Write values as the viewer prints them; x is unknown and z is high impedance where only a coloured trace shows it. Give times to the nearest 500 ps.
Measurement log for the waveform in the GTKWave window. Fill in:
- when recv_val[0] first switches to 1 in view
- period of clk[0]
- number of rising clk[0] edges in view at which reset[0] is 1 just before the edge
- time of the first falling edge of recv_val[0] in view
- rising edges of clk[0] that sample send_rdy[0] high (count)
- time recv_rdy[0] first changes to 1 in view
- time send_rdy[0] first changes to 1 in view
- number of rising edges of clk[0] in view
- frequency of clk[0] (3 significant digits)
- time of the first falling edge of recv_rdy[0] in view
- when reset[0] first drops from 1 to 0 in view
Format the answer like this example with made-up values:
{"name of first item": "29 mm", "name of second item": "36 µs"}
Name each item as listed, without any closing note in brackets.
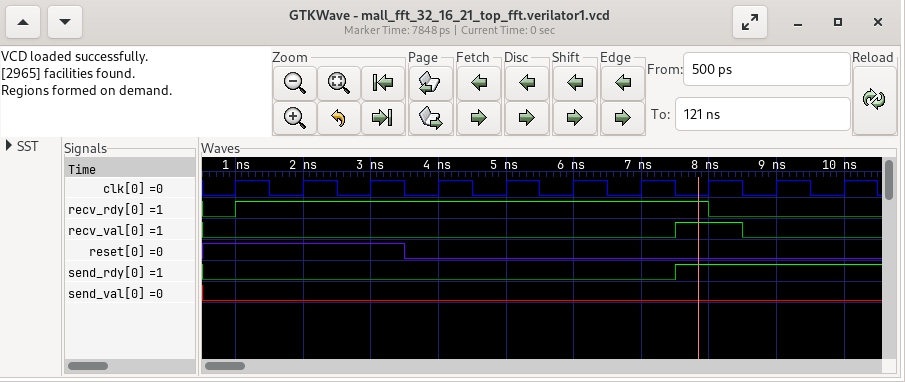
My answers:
{"when recv_val[0] first switches to 1 in view": "7500 ps", "period of clk[0]": "1000 ps", "number of rising clk[0] edges in view at which reset[0] is 1 just before the edge": "3", "time of the first falling edge of recv_val[0] in view": "8500 ps", "rising edges of clk[0] that sample send_rdy[0] high": "3", "time recv_rdy[0] first changes to 1 in view": "1000 ps", "time send_rdy[0] first changes to 1 in view": "7500 ps", "number of rising edges of clk[0] in view": "10", "frequency of clk[0]": "1.00 GHz", "time of the first falling edge of recv_rdy[0] in view": "8000 ps", "when reset[0] first drops from 1 to 0 in view": "3500 ps"}
